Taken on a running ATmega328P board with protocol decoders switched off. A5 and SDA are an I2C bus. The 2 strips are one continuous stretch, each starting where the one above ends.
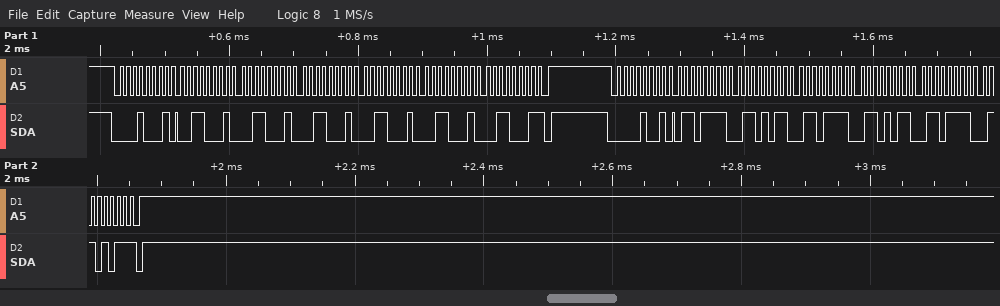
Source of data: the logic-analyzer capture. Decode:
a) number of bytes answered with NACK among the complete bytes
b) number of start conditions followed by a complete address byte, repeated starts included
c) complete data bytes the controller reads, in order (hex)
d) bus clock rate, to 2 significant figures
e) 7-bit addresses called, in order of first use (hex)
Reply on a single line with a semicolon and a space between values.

2; 2; 31 31 31 31 31 31 6F 6B 6F 6B 6F 6B; 100 kHz; 0x08 0x04
